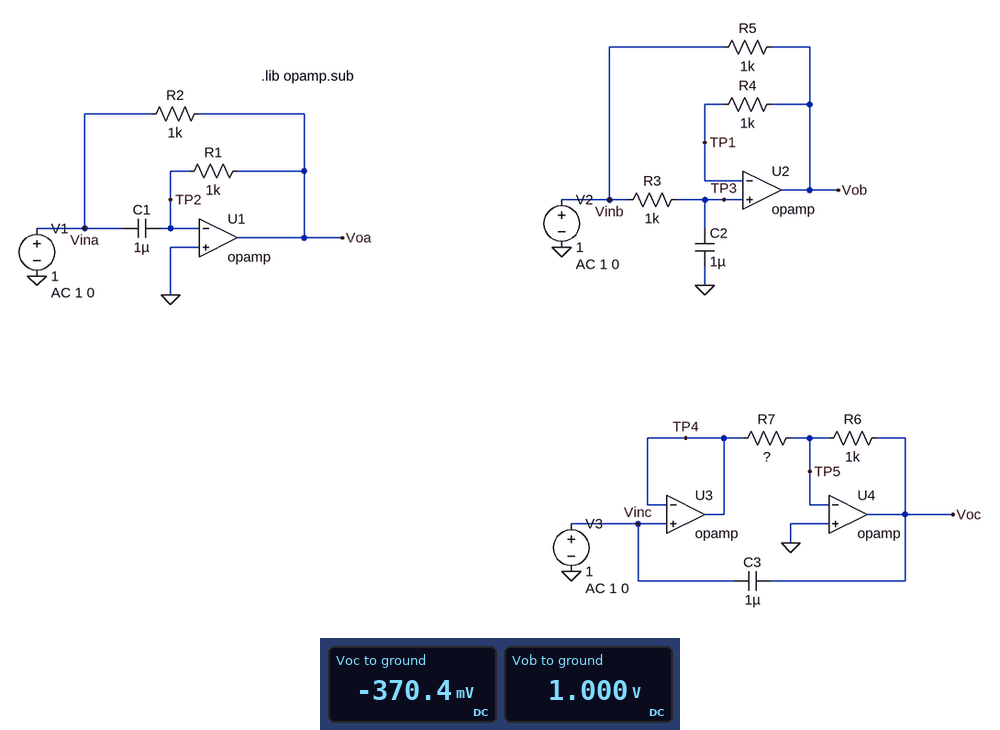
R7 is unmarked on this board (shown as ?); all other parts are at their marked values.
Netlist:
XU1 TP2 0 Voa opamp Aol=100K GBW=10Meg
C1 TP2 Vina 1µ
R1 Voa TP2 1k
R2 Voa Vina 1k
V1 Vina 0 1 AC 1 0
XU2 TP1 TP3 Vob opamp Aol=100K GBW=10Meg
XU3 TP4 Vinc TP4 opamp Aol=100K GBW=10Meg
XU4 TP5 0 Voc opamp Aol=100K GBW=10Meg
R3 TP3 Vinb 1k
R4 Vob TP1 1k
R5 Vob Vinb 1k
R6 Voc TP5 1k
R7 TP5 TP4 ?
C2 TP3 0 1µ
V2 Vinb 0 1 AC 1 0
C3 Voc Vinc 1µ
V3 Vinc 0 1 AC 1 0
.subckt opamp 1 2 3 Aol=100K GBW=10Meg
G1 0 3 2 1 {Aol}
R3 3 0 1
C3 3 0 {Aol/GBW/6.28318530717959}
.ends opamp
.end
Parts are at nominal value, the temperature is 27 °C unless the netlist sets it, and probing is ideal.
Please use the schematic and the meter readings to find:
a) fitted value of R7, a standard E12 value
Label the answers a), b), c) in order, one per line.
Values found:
a) 2.7 kΩ
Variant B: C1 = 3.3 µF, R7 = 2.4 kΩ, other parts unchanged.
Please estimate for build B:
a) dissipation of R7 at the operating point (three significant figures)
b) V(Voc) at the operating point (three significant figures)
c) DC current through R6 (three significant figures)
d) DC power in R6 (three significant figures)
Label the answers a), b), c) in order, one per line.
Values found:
a) 417 µW
b) -417 mV
c) 417 µA
d) 174 µW
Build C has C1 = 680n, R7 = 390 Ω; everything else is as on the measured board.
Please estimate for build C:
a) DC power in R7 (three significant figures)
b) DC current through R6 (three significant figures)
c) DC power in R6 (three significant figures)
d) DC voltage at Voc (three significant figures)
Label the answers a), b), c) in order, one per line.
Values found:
a) 2.56 mW
b) 2.56 mA
c) 6.57 mW
d) -2.56 V
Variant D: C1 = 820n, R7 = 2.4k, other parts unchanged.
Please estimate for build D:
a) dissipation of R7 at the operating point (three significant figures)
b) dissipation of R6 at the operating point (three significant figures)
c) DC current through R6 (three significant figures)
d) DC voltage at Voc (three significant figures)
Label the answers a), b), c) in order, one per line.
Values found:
a) 417 µW
b) 174 µW
c) 417 µA
d) -417 mV
